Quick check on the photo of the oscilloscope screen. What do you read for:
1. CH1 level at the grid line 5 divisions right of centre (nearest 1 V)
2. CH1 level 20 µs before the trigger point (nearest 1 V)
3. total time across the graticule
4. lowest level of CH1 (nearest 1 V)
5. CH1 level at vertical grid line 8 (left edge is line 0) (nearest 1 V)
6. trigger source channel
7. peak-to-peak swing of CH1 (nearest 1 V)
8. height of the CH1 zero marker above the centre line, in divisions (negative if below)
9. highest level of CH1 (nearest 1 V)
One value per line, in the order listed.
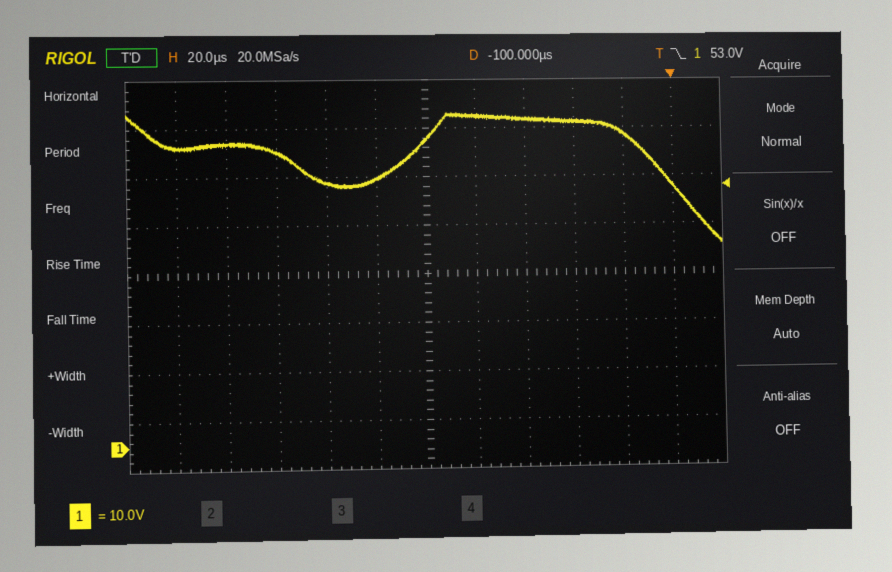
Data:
53 V
64 V
240 µs
41 V
67 V
CH1
27 V
-3.5 div
68 V
